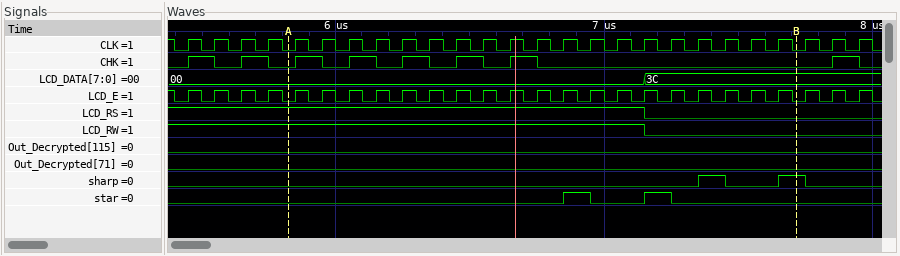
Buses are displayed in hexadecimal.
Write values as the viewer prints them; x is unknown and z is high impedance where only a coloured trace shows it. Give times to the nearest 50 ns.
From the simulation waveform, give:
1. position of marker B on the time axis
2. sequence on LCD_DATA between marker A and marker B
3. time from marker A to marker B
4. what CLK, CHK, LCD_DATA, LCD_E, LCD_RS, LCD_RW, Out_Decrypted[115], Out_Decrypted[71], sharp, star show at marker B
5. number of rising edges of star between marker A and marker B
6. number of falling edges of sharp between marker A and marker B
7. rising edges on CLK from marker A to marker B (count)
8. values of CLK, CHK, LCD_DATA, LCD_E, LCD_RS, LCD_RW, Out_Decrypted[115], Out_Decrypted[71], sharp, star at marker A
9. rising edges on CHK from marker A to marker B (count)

7700 ns
00, 3C
1900 ns
CLK=0, CHK=0, LCD_DATA=3C, LCD_E=0, LCD_RS=0, LCD_RW=0, Out_Decrypted[115]=0, Out_Decrypted[71]=0, sharp=1, star=0
2
1
19
CLK=0, CHK=0, LCD_DATA=00, LCD_E=0, LCD_RS=1, LCD_RW=1, Out_Decrypted[115]=0, Out_Decrypted[71]=0, sharp=0, star=0
5
